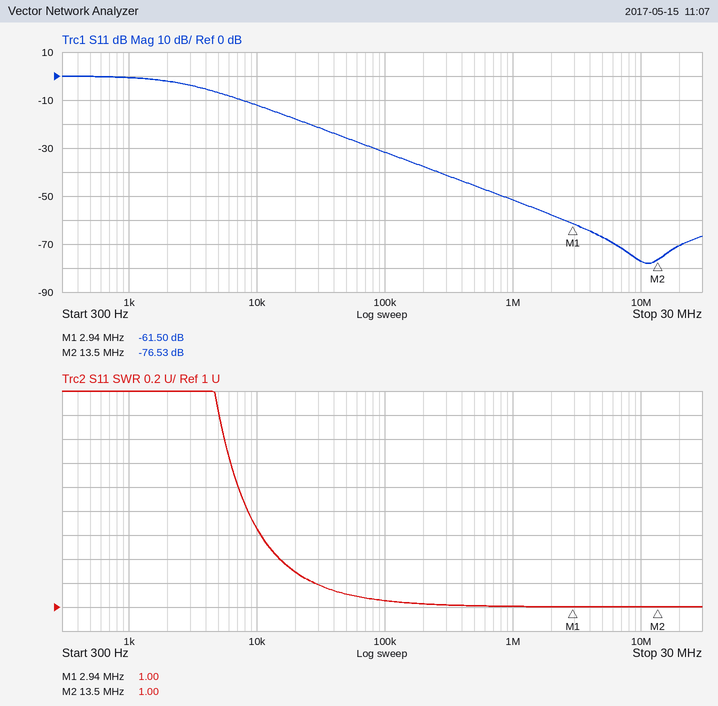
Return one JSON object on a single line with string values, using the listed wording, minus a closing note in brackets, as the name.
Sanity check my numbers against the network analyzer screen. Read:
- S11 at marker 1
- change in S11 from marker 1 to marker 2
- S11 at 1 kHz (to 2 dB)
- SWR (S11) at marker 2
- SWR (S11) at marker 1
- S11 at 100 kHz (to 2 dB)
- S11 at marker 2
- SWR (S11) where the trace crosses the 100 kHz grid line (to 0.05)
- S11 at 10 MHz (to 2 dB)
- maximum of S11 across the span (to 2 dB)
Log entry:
{"S11 at marker 1": "-61.50 dB", "change in S11 from marker 1 to marker 2": "-15.03 dB", "S11 at 1 kHz": "0 dB", "SWR (S11) at marker 2": "1.00", "SWR (S11) at marker 1": "1.00", "S11 at 100 kHz": "-32 dB", "S11 at marker 2": "-76.53 dB", "SWR (S11) where the trace crosses the 100 kHz grid line": "1.05", "S11 at 10 MHz": "-78 dB", "maximum of S11 across the span": "0 dB"}
